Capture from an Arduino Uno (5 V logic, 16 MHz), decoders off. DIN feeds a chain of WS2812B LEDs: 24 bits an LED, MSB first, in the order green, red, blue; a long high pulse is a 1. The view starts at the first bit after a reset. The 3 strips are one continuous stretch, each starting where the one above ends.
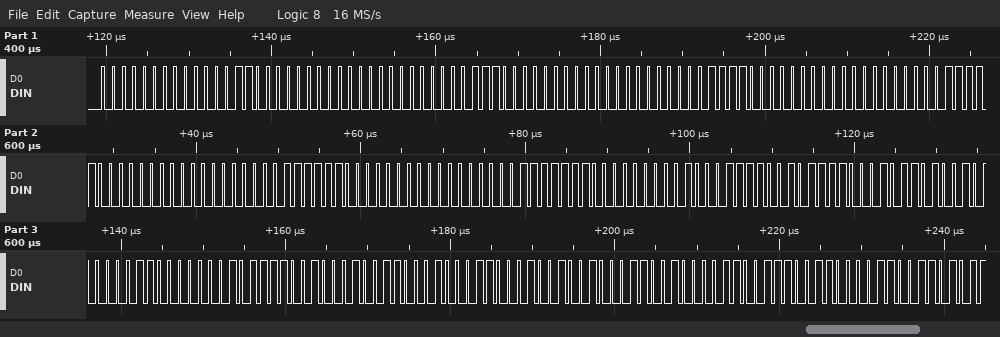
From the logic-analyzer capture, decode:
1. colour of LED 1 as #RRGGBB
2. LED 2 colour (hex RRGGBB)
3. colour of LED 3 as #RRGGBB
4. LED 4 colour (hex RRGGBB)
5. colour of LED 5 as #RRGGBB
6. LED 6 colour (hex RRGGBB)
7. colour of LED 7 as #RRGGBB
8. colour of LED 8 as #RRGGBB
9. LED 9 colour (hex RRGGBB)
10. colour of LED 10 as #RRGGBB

#060000
#0E0000
#1E0000
#3E0000
#7E0000
#FE0000
#2F8F16
#309017
#319118
#329219
